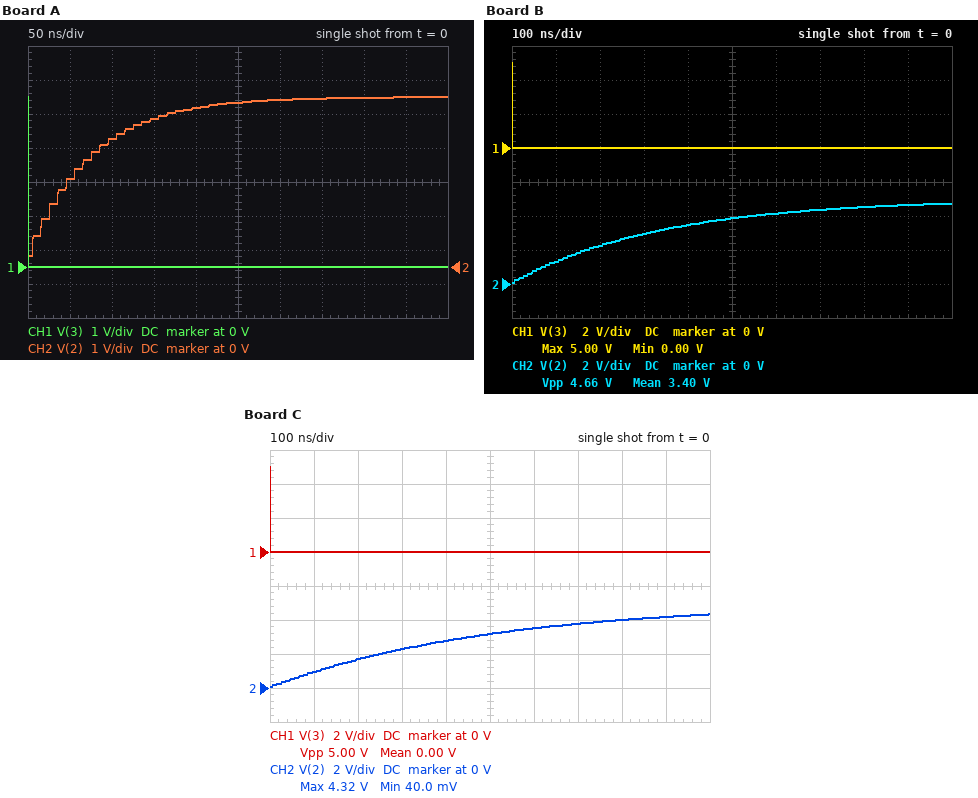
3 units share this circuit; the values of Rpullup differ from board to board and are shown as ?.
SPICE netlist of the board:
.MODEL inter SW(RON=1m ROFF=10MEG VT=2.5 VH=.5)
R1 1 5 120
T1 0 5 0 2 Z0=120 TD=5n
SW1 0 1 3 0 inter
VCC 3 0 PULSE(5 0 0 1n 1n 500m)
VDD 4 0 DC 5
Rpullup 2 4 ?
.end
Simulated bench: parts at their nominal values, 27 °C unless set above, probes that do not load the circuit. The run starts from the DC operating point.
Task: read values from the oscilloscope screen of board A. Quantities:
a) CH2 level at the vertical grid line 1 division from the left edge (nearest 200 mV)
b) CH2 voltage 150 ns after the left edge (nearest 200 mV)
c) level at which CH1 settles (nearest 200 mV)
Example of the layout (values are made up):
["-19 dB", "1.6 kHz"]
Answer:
["2.6 V", "4.4 V", "0 V"]
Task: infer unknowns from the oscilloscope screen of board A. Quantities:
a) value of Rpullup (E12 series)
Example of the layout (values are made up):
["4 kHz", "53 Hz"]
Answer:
["1.8 kΩ"]
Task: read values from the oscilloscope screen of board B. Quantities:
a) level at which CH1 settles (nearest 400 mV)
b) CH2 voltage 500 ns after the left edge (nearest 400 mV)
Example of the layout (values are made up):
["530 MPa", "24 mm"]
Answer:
["0 V", "4.0 V"]
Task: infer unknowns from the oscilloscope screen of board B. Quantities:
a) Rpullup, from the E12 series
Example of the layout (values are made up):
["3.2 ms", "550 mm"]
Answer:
["8.2 kΩ"]
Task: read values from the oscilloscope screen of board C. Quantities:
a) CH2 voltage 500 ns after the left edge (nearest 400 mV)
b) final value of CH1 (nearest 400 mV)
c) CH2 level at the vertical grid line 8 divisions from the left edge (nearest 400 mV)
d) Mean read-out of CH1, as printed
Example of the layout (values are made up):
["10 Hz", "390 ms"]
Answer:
["3.2 V", "0 V", "4.0 V", "0.00 V"]
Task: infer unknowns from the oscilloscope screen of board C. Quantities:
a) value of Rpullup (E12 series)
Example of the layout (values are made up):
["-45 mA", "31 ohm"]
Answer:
["12 kΩ"]
